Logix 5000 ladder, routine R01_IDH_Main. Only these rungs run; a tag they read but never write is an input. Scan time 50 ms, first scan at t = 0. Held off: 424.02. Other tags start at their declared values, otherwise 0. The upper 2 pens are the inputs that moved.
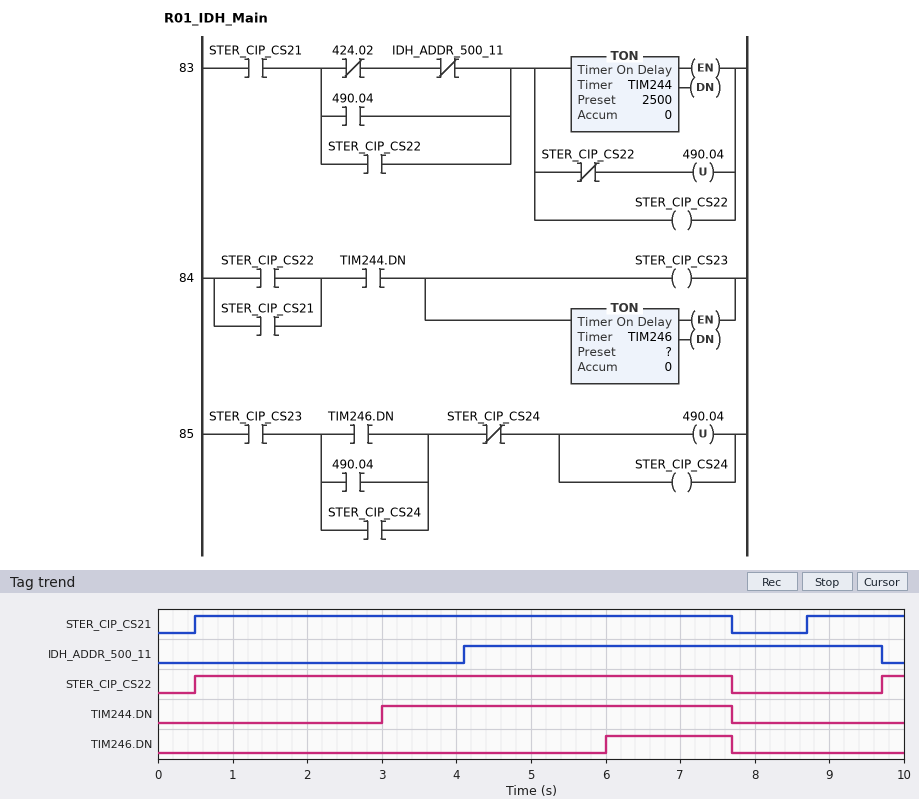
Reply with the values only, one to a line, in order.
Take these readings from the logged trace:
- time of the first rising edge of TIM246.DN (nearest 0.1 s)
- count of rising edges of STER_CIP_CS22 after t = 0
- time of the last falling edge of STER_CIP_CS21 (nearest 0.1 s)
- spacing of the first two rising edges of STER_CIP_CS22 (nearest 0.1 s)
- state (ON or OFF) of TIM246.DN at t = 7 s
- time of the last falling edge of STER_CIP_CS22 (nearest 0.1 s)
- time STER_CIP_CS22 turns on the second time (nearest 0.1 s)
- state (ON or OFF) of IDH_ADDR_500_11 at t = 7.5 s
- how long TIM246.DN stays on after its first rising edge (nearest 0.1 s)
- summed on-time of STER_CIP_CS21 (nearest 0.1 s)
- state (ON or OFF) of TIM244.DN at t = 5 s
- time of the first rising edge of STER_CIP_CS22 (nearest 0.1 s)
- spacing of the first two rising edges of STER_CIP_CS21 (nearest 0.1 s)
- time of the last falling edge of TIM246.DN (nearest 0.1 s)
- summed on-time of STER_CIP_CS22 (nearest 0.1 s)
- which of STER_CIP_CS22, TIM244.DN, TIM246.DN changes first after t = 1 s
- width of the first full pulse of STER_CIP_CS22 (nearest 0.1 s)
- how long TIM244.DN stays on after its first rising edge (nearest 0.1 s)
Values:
6.0 s
2
7.7 s
9.2 s
ON
7.7 s
9.7 s
ON
1.7 s
8.5 s
ON
0.5 s
8.2 s
7.7 s
7.5 s
TIM244.DN
7.2 s
4.7 s
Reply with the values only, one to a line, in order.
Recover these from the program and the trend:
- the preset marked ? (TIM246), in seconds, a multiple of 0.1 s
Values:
3.0 s
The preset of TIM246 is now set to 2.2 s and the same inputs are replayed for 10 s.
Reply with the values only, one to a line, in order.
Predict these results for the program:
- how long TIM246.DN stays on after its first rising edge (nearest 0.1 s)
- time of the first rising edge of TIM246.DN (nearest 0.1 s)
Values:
2.5 s
5.2 s
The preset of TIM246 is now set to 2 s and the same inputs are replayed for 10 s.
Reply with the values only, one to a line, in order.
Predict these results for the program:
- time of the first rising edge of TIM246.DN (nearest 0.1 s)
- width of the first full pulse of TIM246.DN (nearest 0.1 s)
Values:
5.0 s
2.7 s
